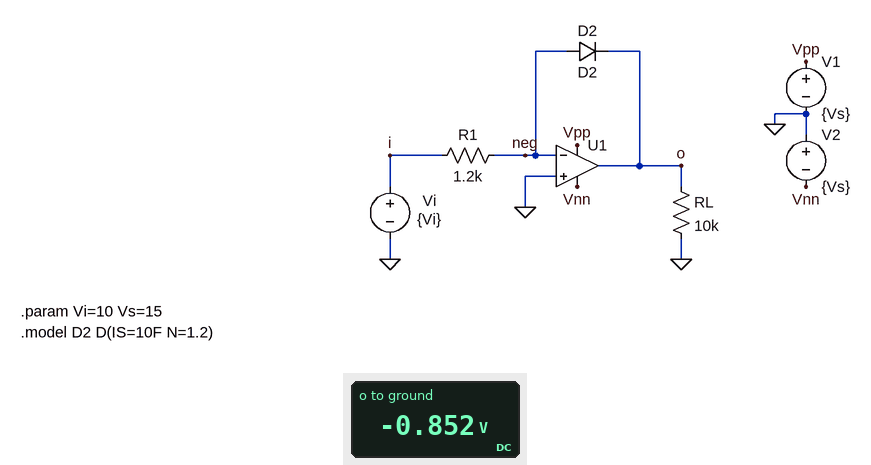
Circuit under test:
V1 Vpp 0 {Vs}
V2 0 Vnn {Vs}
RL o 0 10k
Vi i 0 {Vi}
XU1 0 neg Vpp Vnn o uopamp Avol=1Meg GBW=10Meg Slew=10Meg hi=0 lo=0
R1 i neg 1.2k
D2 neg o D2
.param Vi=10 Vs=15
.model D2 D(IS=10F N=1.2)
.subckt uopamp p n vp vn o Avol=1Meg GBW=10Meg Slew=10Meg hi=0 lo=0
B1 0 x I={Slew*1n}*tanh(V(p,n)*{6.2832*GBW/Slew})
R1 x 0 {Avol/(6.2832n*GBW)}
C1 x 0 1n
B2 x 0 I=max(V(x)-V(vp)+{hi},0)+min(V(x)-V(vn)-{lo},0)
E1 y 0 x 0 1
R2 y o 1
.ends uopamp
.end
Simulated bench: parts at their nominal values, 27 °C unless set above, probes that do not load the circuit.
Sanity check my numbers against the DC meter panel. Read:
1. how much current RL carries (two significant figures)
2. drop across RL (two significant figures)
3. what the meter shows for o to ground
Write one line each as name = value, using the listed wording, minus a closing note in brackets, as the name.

how much current RL carries = 85 µA
drop across RL = 850 mV
what the meter shows for o to ground = -0.852 V
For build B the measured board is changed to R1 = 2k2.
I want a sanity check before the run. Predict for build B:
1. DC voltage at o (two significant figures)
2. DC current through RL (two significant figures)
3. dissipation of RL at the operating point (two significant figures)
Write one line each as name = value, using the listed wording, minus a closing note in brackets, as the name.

DC voltage at o = -830 mV
DC current through RL = 83 µA
dissipation of RL at the operating point = 69 µW
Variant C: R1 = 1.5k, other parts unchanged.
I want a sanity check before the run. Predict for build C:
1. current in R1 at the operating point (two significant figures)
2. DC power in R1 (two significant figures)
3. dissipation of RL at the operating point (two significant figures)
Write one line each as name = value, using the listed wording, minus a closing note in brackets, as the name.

current in R1 at the operating point = 6.7 mA
DC power in R1 = 67 mW
dissipation of RL at the operating point = 71 µW
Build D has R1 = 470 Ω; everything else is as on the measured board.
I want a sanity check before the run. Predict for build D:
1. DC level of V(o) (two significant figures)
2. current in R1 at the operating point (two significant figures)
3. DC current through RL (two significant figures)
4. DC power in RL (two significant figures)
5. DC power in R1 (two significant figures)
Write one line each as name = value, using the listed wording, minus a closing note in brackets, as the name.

DC level of V(o) = -880 mV
current in R1 at the operating point = 21 mA
DC current through RL = 88 µA
DC power in RL = 78 µW
DC power in R1 = 210 mW
